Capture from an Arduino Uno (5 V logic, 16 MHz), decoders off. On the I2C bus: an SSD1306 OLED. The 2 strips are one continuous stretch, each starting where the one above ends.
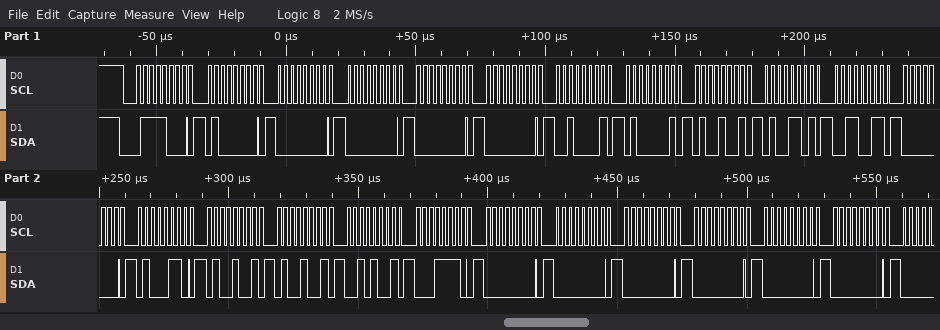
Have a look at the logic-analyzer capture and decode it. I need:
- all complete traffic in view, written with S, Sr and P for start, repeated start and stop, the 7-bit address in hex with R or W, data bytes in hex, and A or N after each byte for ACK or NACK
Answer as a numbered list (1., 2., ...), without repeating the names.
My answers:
1. S 3CW A 40 A 00 A 00 A 00 A 00 A 21 A 41 A 49 A 4D A 33 A 00 A 46 A 49 A 49 A 29 A 1E A 00 A 00 A 00 A 00 A 00 A 00 A
